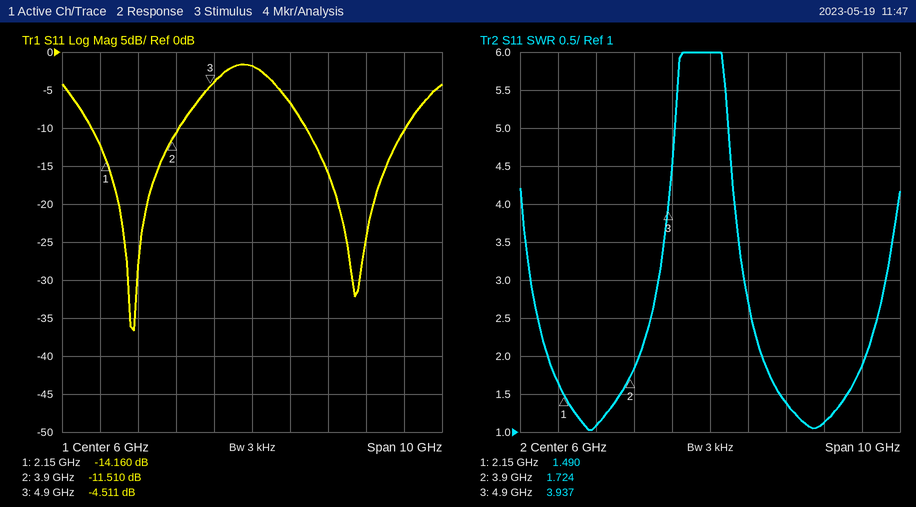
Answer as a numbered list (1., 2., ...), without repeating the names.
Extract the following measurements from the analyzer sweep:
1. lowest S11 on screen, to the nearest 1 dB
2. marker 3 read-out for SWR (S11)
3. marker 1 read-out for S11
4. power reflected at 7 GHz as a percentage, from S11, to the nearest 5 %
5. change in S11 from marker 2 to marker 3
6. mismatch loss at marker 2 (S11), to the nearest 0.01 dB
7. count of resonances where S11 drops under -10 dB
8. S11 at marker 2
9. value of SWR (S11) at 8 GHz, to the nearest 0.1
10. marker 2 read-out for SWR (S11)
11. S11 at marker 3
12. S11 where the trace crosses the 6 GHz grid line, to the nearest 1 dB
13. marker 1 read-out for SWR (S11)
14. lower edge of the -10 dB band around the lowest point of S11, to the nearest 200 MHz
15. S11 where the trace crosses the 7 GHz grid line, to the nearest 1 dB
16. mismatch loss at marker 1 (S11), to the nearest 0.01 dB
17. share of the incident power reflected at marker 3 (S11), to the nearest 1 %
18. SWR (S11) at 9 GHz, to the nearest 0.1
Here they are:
1. -37 dB
2. 3.937
3. -14.160 dB
4. 20 %
5. 6.999 dB
6. 0.32 dB
7. 2
8. -11.510 dB
9. 1.4
10. 1.724
11. -4.511 dB
12. -2 dB
13. 1.490
14. 1.8 GHz
15. -7 dB
16. 0.17 dB
17. 35 %
18. 1.1
